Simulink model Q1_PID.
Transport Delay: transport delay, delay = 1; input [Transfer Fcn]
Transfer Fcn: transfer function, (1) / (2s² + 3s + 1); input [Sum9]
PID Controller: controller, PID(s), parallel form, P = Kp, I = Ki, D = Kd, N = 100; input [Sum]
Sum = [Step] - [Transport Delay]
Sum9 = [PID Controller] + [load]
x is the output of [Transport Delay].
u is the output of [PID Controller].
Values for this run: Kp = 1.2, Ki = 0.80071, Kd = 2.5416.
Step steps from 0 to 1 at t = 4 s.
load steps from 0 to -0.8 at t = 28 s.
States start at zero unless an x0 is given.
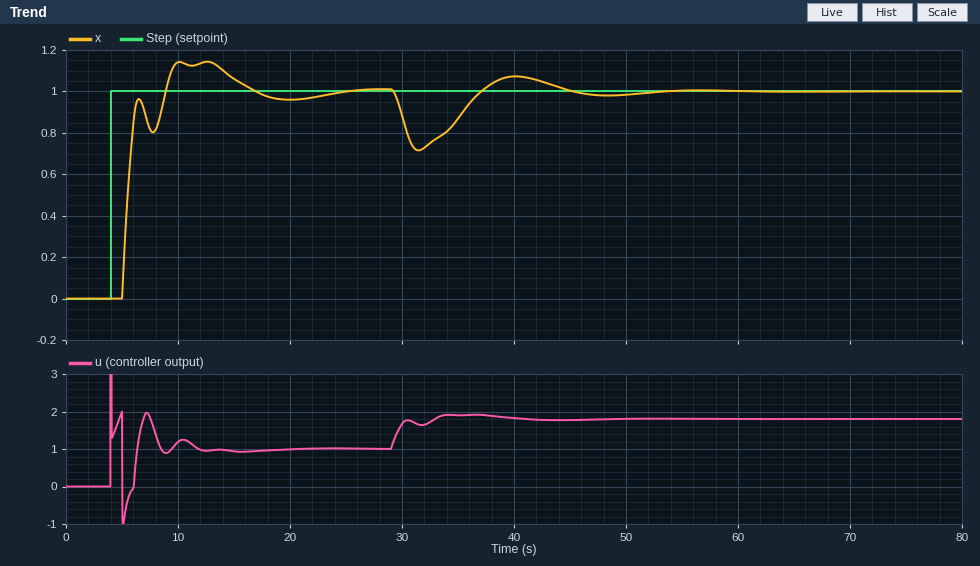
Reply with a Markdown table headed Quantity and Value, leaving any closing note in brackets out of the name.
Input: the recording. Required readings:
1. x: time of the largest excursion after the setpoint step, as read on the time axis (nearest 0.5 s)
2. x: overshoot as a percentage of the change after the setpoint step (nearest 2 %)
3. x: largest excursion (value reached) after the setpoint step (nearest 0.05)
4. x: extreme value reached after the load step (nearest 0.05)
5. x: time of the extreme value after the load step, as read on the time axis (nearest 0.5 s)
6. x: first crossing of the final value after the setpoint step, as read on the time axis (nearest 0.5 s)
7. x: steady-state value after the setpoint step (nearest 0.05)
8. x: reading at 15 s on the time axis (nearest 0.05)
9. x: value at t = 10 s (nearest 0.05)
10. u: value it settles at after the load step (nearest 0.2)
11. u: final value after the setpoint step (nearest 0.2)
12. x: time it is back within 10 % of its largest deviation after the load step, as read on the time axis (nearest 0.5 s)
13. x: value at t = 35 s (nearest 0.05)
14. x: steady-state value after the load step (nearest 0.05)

| Quantity | Value |
|---|---|
| x: time of the largest excursion after the setpoint step, as read on the time axis | 12.5 s |
| x: overshoot as a percentage of the change after the setpoint step | 14 % |
| x: largest excursion (value reached) after the setpoint step | 1.15 |
| x: extreme value reached after the load step | 0.70 |
| x: time of the extreme value after the load step, as read on the time axis | 31.5 s |
| x: first crossing of the final value after the setpoint step, as read on the time axis | 9.0 s |
| x: steady-state value after the setpoint step | 1.00 |
| x: reading at 15 s on the time axis | 1.05 |
| x: value at t = 10 s | 1.15 |
| u: value it settles at after the load step | 1.8 |
| u: final value after the setpoint step | 1.0 |
| x: time it is back within 10 % of its largest deviation after the load step, as read on the time axis | 43.5 s |
| x: value at t = 35 s | 0.85 |
| x: steady-state value after the load step | 1.00 |
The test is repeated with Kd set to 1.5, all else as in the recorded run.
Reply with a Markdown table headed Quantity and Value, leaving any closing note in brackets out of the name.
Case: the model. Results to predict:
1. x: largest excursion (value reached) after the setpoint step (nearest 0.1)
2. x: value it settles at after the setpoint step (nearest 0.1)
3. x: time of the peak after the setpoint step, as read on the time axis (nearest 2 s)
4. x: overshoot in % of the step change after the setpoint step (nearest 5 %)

| Quantity | Value |
|---|---|
| x: largest excursion (value reached) after the setpoint step | 1.2 |
| x: value it settles at after the setpoint step | 1.0 |
| x: time of the peak after the setpoint step, as read on the time axis | 10 s |
| x: overshoot in % of the step change after the setpoint step | 20 % |
